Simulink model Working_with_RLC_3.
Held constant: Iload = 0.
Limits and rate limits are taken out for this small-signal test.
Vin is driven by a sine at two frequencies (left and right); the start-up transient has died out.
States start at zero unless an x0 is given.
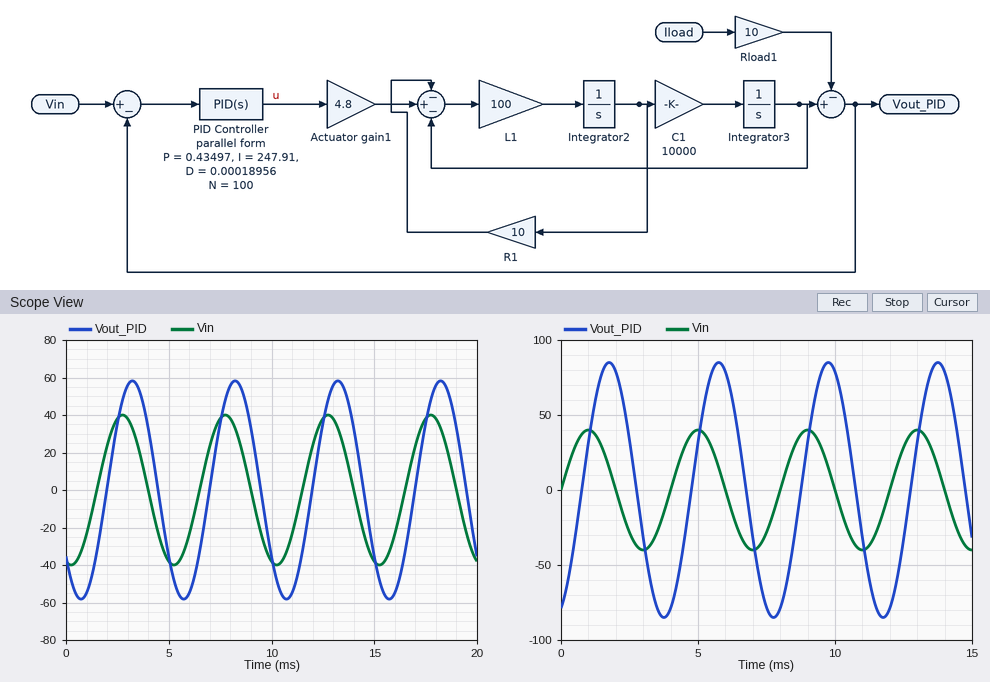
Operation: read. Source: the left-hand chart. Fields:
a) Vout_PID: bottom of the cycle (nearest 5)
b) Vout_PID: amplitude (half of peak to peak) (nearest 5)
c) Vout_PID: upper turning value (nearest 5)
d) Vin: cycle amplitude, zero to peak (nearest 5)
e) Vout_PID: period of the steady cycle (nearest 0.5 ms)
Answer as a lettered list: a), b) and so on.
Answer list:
a) -60
b) 60
c) 60
d) 40
e) 5.0 ms
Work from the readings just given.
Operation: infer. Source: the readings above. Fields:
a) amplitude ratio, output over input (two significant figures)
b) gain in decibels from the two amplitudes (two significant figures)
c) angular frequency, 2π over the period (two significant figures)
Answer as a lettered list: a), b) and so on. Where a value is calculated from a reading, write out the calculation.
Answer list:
a) 60 / 40 = 1.5
b) 20 log10(60 / 40) = 3.5 dB
c) 2π / 5 = 1.3 rad/ms
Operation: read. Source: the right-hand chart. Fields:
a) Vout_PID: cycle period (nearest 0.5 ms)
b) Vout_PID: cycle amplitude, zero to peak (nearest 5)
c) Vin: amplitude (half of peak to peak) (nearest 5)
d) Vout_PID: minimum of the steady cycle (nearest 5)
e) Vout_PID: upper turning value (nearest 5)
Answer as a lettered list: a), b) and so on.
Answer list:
a) 4.0 ms
b) 85
c) 40
d) -85
e) 85
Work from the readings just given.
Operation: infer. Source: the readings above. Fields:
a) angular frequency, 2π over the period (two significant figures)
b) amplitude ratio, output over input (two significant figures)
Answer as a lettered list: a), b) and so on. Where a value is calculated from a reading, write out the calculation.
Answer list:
a) 2π / 4 = 1.6 rad/ms
b) 85 / 40 = 2.1
